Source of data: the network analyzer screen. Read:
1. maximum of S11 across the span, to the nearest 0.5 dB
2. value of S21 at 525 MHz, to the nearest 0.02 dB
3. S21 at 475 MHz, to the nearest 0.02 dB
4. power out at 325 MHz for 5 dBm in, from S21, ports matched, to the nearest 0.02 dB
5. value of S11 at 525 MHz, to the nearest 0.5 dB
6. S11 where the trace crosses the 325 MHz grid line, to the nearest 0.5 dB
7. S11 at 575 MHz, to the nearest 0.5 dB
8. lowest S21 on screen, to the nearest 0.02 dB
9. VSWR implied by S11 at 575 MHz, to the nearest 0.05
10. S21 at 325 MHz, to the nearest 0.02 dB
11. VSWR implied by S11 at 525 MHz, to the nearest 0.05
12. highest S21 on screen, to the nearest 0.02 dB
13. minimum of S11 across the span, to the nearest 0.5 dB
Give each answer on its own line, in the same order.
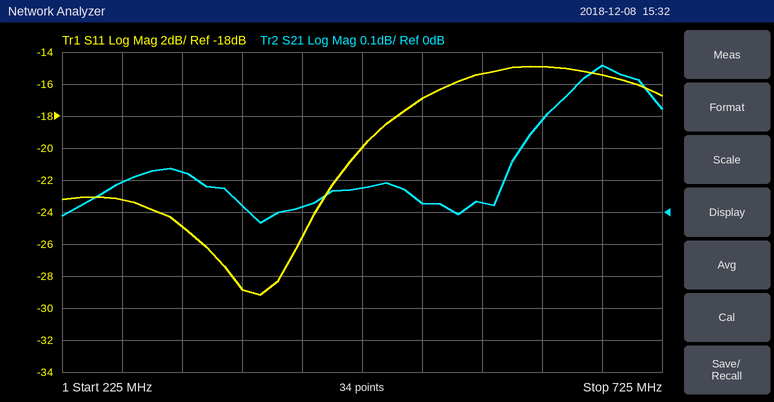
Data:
-15.0 dB
0.02 dB
0.08 dB
5.12 dBm
-17.0 dB
-25.0 dB
-15.5 dB
-0.04 dB
1.40
0.12 dB
1.35
0.46 dB
-29.0 dB
